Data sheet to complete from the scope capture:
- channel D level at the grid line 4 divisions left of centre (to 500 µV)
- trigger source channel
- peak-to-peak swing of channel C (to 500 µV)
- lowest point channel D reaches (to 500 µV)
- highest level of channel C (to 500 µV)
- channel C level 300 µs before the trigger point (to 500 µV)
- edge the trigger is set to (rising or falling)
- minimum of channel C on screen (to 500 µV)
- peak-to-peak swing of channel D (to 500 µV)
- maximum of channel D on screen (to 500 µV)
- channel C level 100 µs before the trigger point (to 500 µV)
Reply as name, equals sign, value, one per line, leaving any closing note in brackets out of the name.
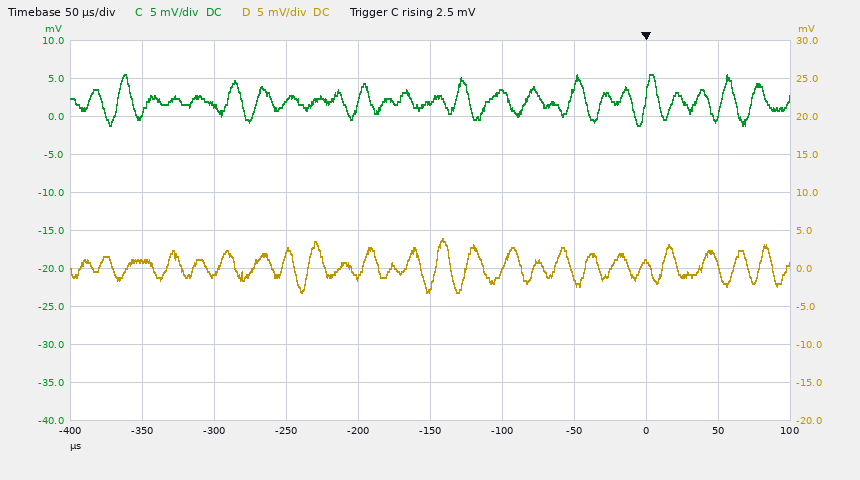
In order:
channel D level at the grid line 4 divisions left of centre = 1.0 mV
trigger source channel = channel C
peak-to-peak swing of channel C = 6.5 mV
lowest point channel D reaches = -3.0 mV
highest level of channel C = 5.5 mV
channel C level 300 µs before the trigger point = 1.5 mV
edge the trigger is set to = rising
minimum of channel C on screen = -1.0 mV
peak-to-peak swing of channel D = 7.0 mV
maximum of channel D on screen = 4.0 mV
channel C level 100 µs before the trigger point = 3.5 mV
